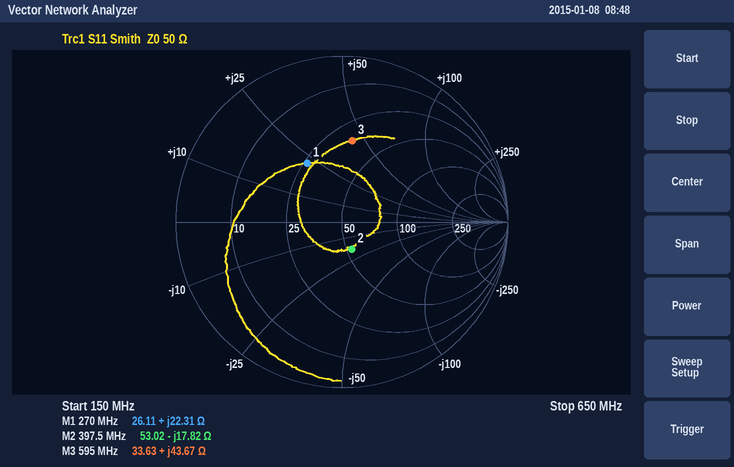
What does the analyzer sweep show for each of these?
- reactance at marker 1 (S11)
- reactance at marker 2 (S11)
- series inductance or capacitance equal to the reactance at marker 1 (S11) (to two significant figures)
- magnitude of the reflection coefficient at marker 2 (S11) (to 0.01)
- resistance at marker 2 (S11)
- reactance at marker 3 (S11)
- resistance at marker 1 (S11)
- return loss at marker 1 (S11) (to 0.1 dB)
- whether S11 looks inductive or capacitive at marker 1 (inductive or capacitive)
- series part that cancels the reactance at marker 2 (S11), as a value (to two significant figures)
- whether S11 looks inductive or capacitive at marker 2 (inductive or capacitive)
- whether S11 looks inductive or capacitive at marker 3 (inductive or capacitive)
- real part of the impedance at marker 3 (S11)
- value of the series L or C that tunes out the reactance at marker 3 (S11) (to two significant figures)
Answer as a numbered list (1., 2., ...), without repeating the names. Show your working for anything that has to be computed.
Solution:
1. +22.31 Ω
2. -17.82 Ω
3. L = 22.31 Ω/(2π × 270 MHz) ≈ 13 nH
4. 0.17
5. 53.02 Ω
6. +43.67 Ω
7. 26.11 Ω
8. 7.7 dB
9. inductive
10. L = 17.82 Ω/(2π × 397.5 MHz) ≈ 7.1 nH
11. capacitive
12. inductive
13. 33.63 Ω
14. C = 1/(2π × 595 MHz × 43.67 Ω) ≈ 6.1 pF
